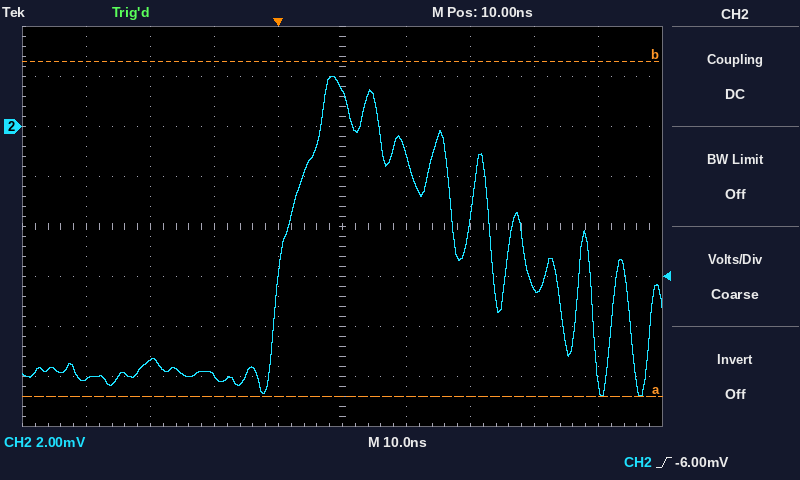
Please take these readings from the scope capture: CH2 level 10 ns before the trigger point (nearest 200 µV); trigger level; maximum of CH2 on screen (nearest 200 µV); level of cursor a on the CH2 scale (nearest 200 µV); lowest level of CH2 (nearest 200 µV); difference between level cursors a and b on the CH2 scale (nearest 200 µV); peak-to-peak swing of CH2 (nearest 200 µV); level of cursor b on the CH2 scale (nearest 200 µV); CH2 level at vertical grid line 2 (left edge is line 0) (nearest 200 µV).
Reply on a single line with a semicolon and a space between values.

-10.0 mV; -6.00 mV; 2.0 mV; -10.8 mV; -10.8 mV; 13.4 mV; 12.8 mV; 2.6 mV; -9.4 mV
